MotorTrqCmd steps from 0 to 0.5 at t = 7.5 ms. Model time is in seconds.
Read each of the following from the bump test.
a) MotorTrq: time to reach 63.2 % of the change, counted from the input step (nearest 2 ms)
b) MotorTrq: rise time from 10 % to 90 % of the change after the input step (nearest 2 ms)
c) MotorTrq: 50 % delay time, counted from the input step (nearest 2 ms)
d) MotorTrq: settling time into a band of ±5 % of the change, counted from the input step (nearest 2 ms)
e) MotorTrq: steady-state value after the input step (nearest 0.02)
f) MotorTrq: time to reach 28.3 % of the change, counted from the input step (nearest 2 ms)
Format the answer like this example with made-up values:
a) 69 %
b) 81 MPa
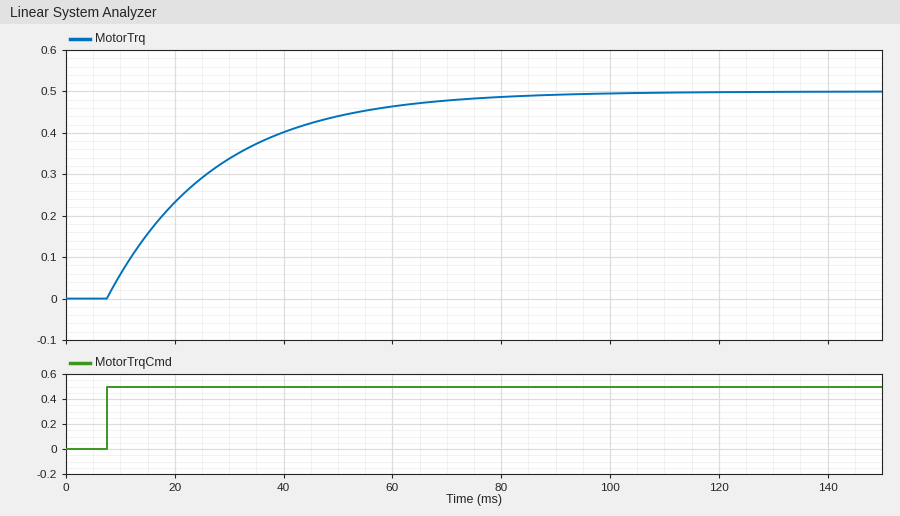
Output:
a) 20 ms
b) 44 ms
c) 14 ms
d) 60 ms
e) 0.50
f) 6 ms
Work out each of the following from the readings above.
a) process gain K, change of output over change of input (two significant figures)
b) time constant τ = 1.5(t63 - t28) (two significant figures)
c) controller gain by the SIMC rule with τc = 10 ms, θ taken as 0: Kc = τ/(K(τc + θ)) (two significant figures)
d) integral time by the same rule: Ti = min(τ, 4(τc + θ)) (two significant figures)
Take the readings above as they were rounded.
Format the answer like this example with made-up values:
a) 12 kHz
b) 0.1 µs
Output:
a) 1.0
b) 21 ms
c) 2.1
d) 21 ms
